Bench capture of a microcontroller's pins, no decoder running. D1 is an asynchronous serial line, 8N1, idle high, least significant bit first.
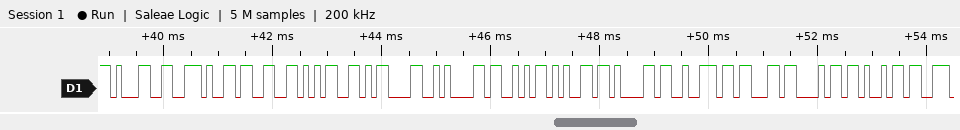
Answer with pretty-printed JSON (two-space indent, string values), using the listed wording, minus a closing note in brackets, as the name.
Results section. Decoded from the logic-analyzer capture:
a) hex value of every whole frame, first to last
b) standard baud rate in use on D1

{
  "hex value of every whole frame, first to last": "0x31 0x2E 0x33 0x35 0x0D 0x0A 0x53 0x65 0x61 0x72 0x63 0x68 0x69",
  "standard baud rate in use on D1": "9600 baud"
}
